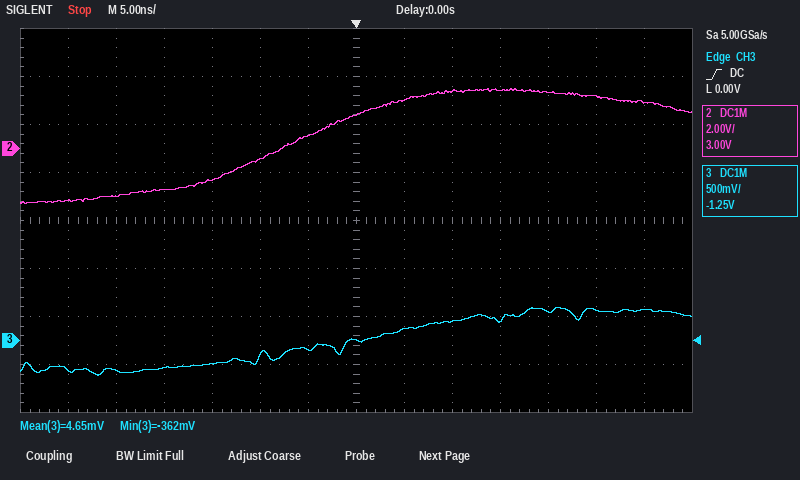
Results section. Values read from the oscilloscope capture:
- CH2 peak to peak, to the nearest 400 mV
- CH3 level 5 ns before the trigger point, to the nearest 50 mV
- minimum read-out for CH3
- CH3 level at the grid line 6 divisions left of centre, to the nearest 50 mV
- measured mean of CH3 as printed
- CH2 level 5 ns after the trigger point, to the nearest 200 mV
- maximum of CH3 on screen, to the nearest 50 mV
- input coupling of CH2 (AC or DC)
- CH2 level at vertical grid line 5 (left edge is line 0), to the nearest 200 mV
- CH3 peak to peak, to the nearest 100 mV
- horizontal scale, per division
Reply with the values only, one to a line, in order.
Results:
4.8 V
-100 mV
-362 mV
-300 mV
4.65 mV
2.0 V
350 mV
DC
-400 mV
700 mV
5 ns
